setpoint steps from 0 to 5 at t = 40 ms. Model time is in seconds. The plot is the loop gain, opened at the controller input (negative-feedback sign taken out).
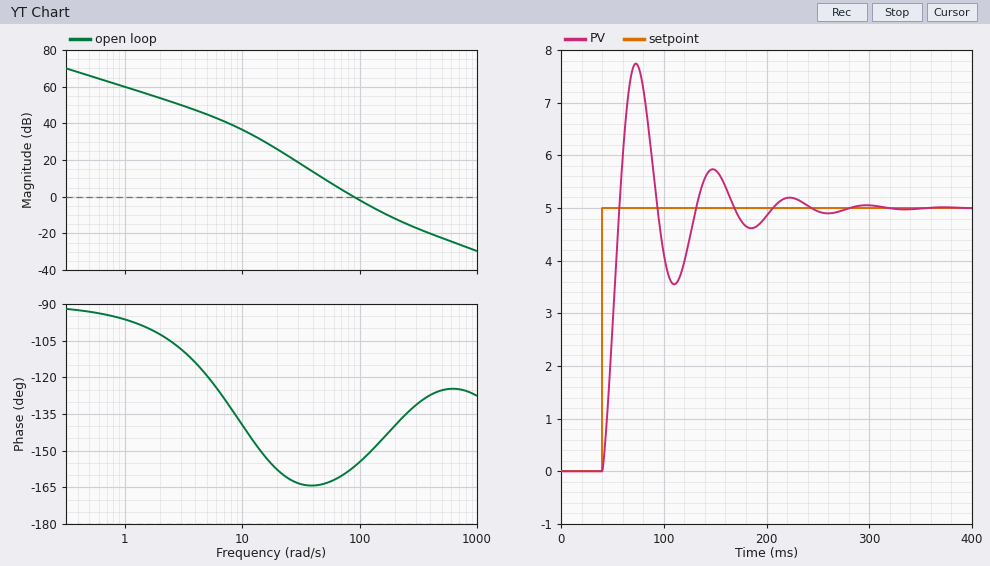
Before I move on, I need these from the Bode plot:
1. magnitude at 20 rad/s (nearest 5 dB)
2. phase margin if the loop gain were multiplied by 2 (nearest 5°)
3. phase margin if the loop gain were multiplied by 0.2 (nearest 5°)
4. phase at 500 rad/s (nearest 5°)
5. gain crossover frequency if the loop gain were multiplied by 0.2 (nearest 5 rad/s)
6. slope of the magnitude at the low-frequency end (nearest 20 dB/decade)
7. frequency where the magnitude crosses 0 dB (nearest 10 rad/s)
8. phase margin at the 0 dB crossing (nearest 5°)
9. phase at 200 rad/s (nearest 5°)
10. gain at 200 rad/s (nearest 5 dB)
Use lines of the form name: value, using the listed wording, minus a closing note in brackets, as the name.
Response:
magnitude at 20 rad/s: 25 dB
phase margin if the loop gain were multiplied by 2: 30°
phase margin if the loop gain were multiplied by 0.2: 15°
phase at 500 rad/s: -125°
gain crossover frequency if the loop gain were multiplied by 0.2: 40 rad/s
slope of the magnitude at the low-frequency end: -20 dB/decade
frequency where the magnitude crosses 0 dB: 90 rad/s
phase margin at the 0 dB crossing: 25°
phase at 200 rad/s: -140°
gain at 200 rad/s: -10 dB
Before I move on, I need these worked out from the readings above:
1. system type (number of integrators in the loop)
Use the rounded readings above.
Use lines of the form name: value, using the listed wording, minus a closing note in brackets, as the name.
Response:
system type: 1
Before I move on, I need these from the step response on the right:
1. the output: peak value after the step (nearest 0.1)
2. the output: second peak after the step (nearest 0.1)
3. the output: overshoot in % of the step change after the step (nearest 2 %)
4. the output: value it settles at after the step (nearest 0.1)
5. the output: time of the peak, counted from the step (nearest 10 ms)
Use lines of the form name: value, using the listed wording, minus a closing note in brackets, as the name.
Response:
the output: peak value after the step: 7.7
the output: second peak after the step: 5.7
the output: overshoot in % of the step change after the step: 54 %
the output: value it settles at after the step: 5.0
the output: time of the peak, counted from the step: 30 ms
